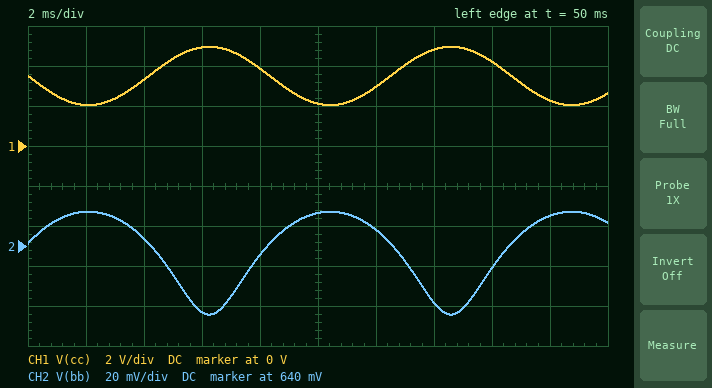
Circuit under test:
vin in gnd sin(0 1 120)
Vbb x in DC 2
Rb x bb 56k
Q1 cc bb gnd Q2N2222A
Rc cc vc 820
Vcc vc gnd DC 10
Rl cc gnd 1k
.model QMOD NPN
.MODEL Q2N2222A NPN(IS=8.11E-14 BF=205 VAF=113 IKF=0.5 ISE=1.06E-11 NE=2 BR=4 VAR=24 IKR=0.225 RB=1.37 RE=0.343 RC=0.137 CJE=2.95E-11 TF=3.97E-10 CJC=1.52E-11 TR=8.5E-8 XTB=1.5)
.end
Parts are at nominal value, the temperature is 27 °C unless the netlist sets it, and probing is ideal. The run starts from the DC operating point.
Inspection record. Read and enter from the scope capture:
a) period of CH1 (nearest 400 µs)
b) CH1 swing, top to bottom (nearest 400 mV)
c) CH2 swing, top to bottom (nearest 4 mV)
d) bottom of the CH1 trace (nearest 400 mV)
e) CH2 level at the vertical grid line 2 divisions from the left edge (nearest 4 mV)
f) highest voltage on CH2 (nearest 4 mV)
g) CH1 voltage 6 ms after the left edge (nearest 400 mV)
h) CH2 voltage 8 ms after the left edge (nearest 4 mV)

8.4 ms
2.8 V
52 mV
2.0 V
644 mV
656 mV
4.8 V
636 mV
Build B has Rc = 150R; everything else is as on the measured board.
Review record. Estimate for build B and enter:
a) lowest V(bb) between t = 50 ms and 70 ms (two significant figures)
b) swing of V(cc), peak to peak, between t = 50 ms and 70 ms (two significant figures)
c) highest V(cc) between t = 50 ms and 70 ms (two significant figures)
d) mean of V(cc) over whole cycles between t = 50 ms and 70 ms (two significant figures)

610 mV
890 mV
8.5 V
8.1 V
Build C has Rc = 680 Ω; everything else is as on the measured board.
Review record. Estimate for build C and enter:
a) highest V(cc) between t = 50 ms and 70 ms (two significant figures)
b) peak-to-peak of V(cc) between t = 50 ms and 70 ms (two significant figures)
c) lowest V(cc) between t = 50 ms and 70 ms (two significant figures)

5.5 V
2.6 V
2.8 V
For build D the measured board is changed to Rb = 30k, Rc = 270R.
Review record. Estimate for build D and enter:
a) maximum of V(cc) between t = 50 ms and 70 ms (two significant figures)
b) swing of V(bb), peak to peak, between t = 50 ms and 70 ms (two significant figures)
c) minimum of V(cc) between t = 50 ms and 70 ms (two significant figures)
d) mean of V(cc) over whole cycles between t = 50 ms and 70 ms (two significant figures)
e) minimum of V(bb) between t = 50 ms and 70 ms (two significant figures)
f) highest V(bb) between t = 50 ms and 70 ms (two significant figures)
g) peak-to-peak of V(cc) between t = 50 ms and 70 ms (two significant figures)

7.4 V
54 mV
4.8 V
6.1 V
620 mV
680 mV
2.6 V
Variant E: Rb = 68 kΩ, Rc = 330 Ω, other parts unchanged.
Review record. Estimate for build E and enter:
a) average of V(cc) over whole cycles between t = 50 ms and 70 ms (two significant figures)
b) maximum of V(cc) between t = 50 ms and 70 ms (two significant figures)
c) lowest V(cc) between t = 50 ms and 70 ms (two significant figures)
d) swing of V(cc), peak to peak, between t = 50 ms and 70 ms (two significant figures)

6.6 V
7.3 V
5.9 V
1.4 V
